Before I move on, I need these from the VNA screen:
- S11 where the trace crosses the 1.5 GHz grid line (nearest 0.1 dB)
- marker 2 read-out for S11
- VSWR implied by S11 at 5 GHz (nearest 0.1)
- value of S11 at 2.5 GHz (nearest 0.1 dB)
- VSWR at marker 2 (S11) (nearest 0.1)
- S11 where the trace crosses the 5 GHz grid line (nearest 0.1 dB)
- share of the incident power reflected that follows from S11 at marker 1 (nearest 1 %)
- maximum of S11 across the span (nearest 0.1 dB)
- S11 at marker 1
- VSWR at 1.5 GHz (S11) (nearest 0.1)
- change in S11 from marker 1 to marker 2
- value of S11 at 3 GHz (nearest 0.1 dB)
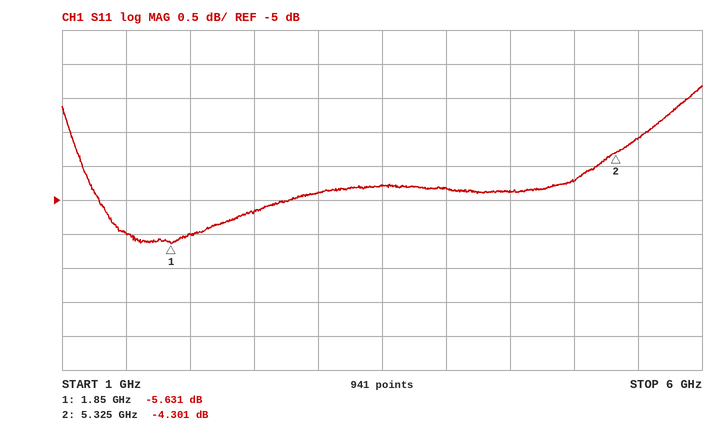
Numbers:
-5.5 dB
-4.301 dB
3.8
-5.2 dB
4.1
-4.7 dB
27 %
-3.3 dB
-5.631 dB
3.3
1.330 dB
-4.9 dB
